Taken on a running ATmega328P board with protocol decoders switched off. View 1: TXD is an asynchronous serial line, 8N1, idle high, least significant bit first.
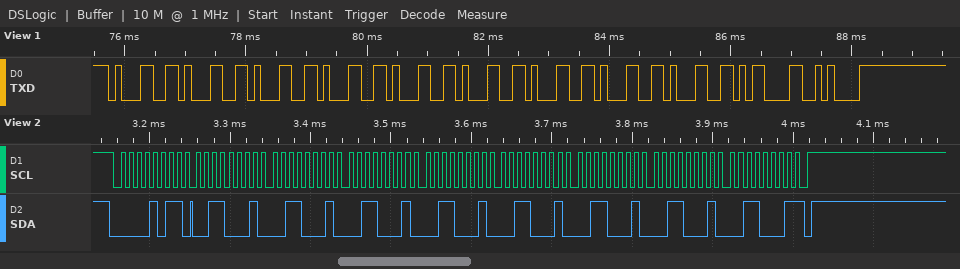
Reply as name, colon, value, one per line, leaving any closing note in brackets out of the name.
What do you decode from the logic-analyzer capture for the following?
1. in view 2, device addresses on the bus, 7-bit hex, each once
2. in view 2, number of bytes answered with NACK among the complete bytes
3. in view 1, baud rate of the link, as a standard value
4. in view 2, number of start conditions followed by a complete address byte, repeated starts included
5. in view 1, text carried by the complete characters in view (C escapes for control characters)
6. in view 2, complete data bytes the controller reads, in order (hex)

in view 2, device addresses on the bus, 7-bit hex, each once: 0x05
in view 2, number of bytes answered with NACK among the complete bytes: 1
in view 1, baud rate of the link, as a standard value: 9600 baud
in view 2, number of start conditions followed by a complete address byte, repeated starts included: 1
in view 1, text carried by the complete characters in view: "111111111\r\n"
in view 2, complete data bytes the controller reads, in order: 31 31 31 31 31 31 31 31
